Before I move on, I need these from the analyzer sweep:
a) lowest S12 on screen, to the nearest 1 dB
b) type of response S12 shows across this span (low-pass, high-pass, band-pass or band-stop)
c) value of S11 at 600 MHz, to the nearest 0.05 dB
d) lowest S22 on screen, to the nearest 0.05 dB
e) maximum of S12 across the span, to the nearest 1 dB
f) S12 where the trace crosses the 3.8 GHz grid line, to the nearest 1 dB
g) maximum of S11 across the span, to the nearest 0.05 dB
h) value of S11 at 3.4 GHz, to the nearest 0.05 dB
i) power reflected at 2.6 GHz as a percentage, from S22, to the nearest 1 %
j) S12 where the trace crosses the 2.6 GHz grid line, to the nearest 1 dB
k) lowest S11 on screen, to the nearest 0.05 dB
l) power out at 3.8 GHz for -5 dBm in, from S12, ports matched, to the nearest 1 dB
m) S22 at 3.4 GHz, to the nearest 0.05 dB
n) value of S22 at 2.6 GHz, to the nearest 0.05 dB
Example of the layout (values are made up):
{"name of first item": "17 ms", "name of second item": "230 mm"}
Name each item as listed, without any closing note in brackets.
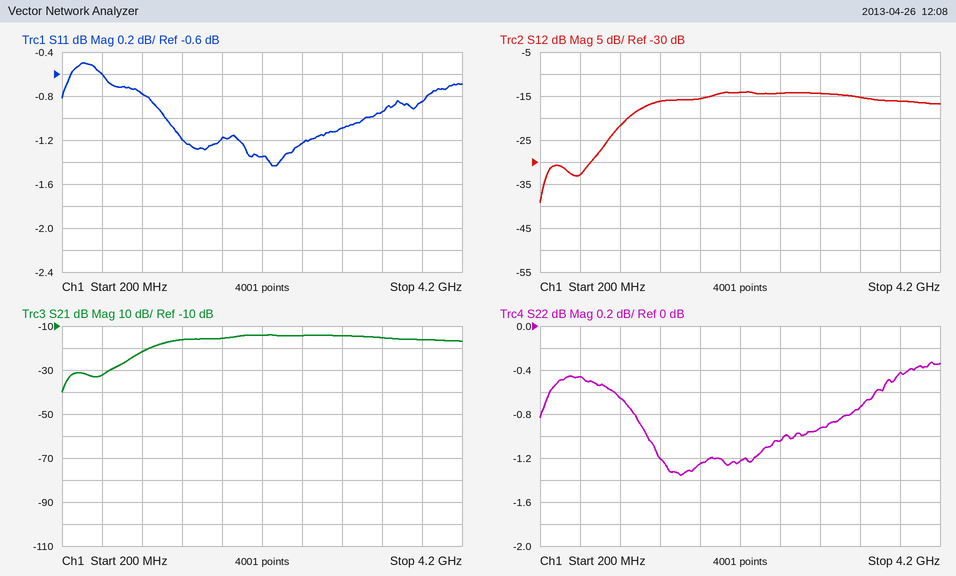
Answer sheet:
{"lowest S12 on screen, to the nearest 1 dB": "-39 dB", "type of response S12 shows across this span": "high-pass", "value of S11 at 600 MHz, to the nearest 0.05 dB": "-0.60 dB", "lowest S22 on screen, to the nearest 0.05 dB": "-1.35 dB", "maximum of S12 across the span, to the nearest 1 dB": "-14 dB", "S12 where the trace crosses the 3.8 GHz grid line, to the nearest 1 dB": "-16 dB", "maximum of S11 across the span, to the nearest 0.05 dB": "-0.50 dB", "value of S11 at 3.4 GHz, to the nearest 0.05 dB": "-0.95 dB", "power reflected at 2.6 GHz as a percentage, from S22, to the nearest 1 %": "79 %", "S12 where the trace crosses the 2.6 GHz grid line, to the nearest 1 dB": "-14 dB", "lowest S11 on screen, to the nearest 0.05 dB": "-1.45 dB", "power out at 3.8 GHz for -5 dBm in, from S12, ports matched, to the nearest 1 dB": "-21 dBm", "S22 at 3.4 GHz, to the nearest 0.05 dB": "-0.75 dB", "value of S22 at 2.6 GHz, to the nearest 0.05 dB": "-1.05 dB"}
